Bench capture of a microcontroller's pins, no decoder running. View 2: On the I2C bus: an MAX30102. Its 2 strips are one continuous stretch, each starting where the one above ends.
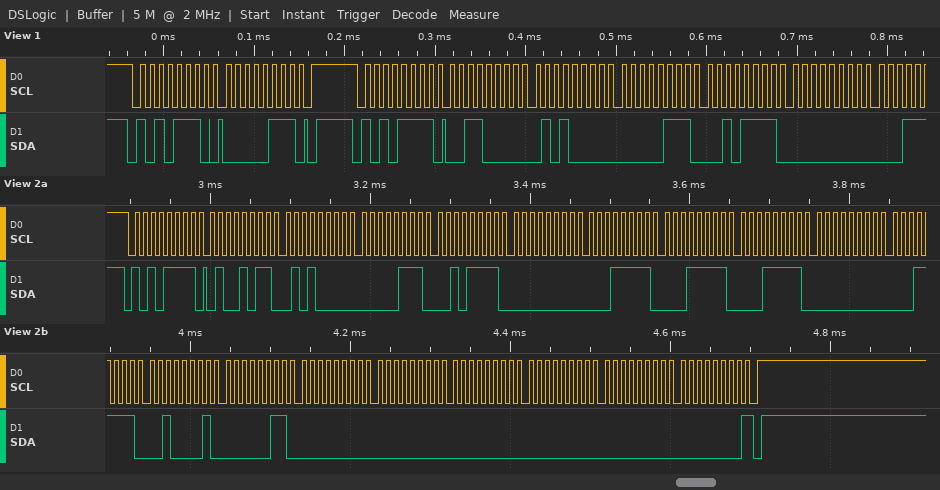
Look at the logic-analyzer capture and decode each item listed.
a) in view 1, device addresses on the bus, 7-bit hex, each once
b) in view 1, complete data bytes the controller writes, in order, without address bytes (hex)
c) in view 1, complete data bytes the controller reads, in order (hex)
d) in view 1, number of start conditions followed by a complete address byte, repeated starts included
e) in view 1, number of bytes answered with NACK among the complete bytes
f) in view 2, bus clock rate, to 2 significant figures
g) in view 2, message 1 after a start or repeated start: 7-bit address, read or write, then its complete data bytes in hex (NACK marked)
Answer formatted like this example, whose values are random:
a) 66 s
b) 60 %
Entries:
a) 0x57
b) 07
c) 30 50 07 2F 00
d) 2
e) 0
f) 100 kHz
g) 0x57 read: 4B 50 07 2F 00 1F 1F 1F 00 1F 21 03 00 00 00 00 00 00 NACK
